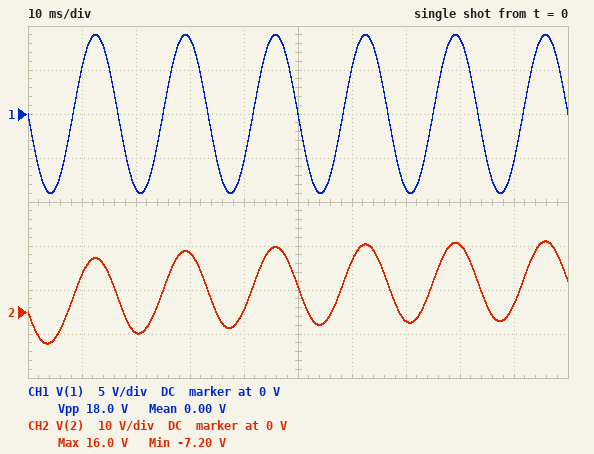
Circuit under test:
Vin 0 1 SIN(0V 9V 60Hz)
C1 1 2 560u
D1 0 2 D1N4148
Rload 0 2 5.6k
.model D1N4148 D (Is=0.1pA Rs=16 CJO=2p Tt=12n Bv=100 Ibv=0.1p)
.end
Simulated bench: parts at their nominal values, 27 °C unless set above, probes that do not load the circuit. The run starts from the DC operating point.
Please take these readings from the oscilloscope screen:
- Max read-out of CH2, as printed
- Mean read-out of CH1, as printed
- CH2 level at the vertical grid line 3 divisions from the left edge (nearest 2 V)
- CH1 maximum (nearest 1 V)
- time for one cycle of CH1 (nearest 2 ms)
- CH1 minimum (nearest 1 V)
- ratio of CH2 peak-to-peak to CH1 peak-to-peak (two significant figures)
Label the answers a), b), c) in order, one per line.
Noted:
a) 16.0 V
b) 0.00 V
c) 14 V
d) 9 V
e) 16 ms
f) -9 V
g) 1.3
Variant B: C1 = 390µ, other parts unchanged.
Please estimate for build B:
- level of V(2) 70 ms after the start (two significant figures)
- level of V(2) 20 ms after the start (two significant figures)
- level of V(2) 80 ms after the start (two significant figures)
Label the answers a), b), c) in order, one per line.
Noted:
a) -1.6 V
b) -3.9 V
c) 16 V
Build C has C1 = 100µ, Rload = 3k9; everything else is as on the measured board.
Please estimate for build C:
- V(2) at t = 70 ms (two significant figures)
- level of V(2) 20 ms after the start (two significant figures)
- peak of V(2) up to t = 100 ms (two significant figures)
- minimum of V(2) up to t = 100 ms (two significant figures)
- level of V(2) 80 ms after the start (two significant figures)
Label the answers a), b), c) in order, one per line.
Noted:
a) -890 mV
b) -1.5 V
c) 17 V
d) -4.0 V
e) 16 V
